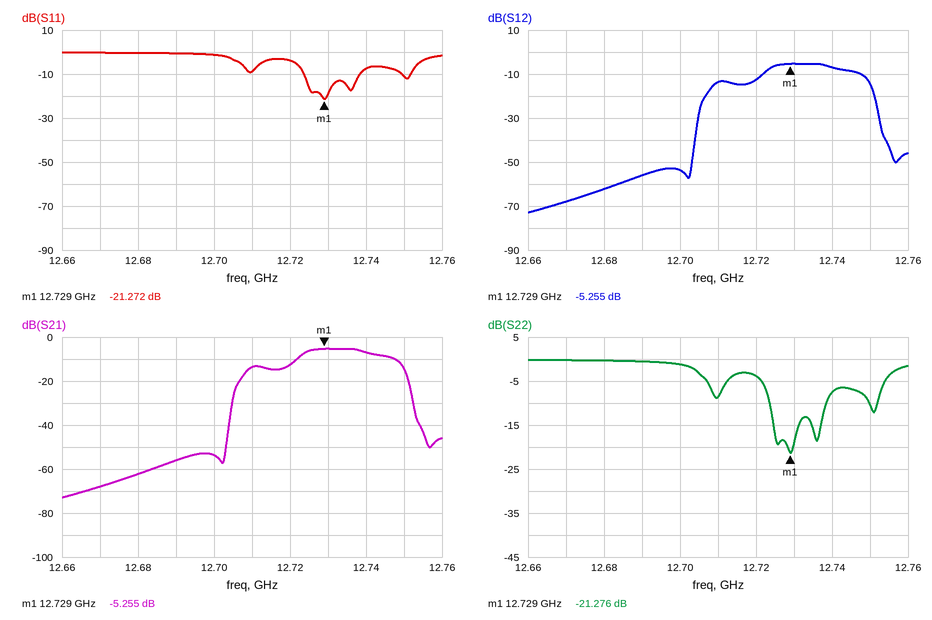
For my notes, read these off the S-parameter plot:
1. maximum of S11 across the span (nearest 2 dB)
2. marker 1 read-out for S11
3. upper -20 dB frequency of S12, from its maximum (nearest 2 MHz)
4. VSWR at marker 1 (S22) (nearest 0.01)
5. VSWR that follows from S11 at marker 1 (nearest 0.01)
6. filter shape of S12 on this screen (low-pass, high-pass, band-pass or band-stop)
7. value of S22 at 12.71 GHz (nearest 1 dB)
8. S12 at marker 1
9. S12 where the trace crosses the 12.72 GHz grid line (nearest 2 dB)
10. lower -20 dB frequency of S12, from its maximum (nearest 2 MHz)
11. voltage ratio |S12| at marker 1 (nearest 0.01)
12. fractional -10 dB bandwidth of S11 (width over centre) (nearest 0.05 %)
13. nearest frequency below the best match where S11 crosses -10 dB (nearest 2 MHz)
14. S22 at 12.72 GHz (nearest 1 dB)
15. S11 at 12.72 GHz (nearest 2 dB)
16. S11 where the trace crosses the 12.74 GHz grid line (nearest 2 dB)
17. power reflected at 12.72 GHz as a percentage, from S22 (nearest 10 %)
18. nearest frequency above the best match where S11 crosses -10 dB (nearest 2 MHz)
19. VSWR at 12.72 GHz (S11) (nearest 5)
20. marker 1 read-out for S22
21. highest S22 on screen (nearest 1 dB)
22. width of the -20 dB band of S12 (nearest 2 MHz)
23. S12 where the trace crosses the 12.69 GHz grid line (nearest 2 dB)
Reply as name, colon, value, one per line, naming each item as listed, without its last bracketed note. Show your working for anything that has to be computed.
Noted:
maximum of S11 across the span: 0 dB
marker 1 read-out for S11: -21.272 dB
upper -20 dB frequency of S12, from its maximum: 12.752 GHz
VSWR at marker 1 (S22): (1 + 0.0863)/(1 − 0.0863) ≈ 1.19
VSWR that follows from S11 at marker 1: (1 + 0.0864)/(1 − 0.0864) ≈ 1.19
filter shape of S12 on this screen: band-pass
value of S22 at 12.71 GHz: -9 dB
S12 at marker 1: -5.255 dB
S12 where the trace crosses the 12.72 GHz grid line: -12 dB
lower -20 dB frequency of S12, from its maximum: 12.706 GHz
voltage ratio |S12| at marker 1: 10^(-5.255/20) ≈ 0.55
fractional -10 dB bandwidth of S11 (width over centre): 14 MHz / 12.731 GHz ≈ 0.110 %, so 0.10 % to the nearest 0.05 %
nearest frequency below the best match where S11 crosses -10 dB: 12.724 GHz
S22 at 12.72 GHz: -4 dB
S11 at 12.72 GHz: -4 dB
S11 where the trace crosses the 12.74 GHz grid line: -8 dB
power reflected at 12.72 GHz as a percentage, from S22: 10^(-4/10) ≈ 40 %
nearest frequency above the best match where S11 crosses -10 dB: 12.738 GHz
VSWR at 12.72 GHz (S11): |Γ| = 10^(-4/20) = 0.6310; VSWR = (1 + 0.6310)/(1 − 0.6310) ≈ 4.42, so 5 to the nearest 5
marker 1 read-out for S22: -21.276 dB
highest S22 on screen: 0 dB
width of the -20 dB band of S12: 12.752 GHz − 12.706 GHz = 46 MHz
S12 where the trace crosses the 12.69 GHz grid line: -56 dB
